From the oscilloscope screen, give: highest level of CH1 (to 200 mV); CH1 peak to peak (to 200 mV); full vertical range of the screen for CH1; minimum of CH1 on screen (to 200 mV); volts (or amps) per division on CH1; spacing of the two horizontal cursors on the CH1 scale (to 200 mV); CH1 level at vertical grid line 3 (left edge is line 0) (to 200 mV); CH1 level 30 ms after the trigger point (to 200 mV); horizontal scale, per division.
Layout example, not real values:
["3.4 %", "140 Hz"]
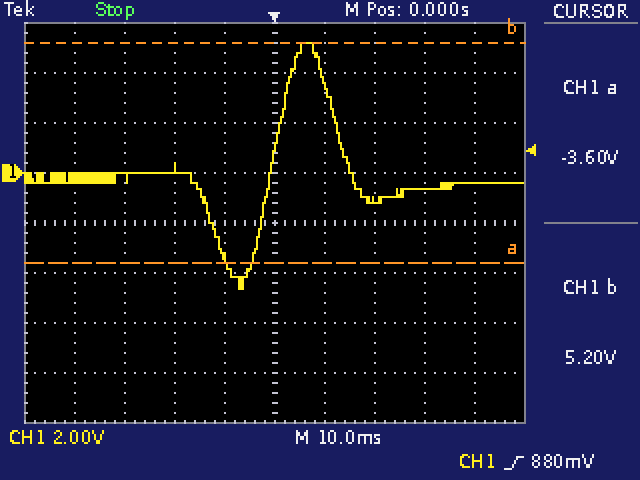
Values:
["5.2 V", "9.8 V", "16 V", "-4.6 V", "2 V", "8.8 V", "200 mV", "-600 mV", "10 ms"]
